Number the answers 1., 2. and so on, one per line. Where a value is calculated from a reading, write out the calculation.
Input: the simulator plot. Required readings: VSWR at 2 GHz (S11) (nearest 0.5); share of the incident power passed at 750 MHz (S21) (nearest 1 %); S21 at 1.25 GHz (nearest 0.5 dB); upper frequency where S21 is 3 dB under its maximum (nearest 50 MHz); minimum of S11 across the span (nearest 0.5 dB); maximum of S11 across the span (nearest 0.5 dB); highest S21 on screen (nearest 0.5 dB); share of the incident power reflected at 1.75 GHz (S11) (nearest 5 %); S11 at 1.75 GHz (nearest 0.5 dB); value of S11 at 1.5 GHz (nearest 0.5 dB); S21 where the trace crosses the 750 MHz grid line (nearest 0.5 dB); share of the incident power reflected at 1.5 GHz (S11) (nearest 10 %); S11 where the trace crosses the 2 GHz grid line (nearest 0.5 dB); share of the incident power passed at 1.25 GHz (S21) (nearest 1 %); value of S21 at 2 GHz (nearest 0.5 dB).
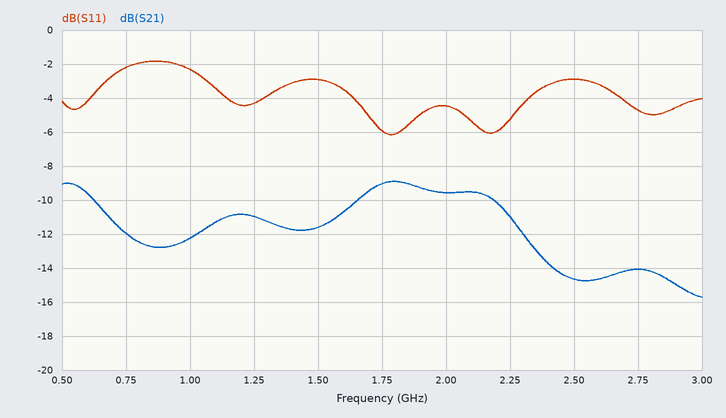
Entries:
1. |Γ| = 10^(-4.5/20) = 0.5957; VSWR = (1 + 0.5957)/(1 − 0.5957) ≈ 4.0
2. 10^(-12/10) ≈ 6 %
3. -11.0 dB
4. 2.30 GHz
5. -6.0 dB
6. -2.0 dB
7. -9.0 dB
8. 10^(-6/10) ≈ 25 %
9. -6.0 dB
10. -3.0 dB
11. -12.0 dB
12. 10^(-3/10) ≈ 50 %
13. -4.5 dB
14. 10^(-11/10) ≈ 8 %
15. -9.5 dB
